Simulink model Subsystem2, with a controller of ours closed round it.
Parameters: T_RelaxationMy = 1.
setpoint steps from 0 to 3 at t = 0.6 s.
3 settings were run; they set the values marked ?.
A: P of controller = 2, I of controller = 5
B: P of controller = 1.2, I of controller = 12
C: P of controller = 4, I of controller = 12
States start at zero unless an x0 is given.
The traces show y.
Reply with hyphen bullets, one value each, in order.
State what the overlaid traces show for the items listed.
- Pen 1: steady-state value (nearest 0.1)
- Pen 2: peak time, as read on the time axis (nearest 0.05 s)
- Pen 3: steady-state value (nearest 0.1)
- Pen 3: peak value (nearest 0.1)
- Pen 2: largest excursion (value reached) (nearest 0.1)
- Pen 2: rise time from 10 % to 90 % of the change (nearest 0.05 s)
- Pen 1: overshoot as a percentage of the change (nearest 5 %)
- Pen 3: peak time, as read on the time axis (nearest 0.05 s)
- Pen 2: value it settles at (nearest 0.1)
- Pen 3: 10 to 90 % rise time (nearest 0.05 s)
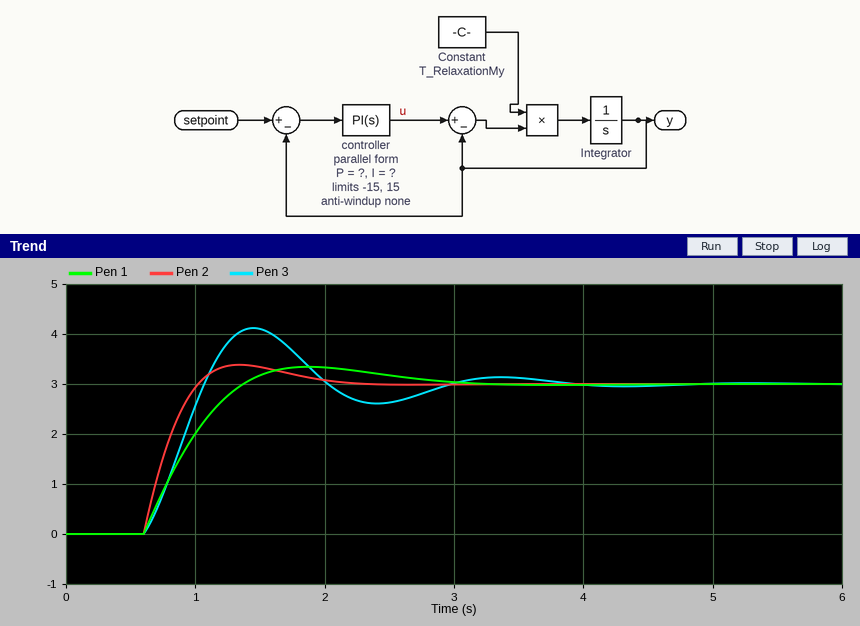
- 3.0
- 1.35 s
- 3.0
- 4.1
- 3.4
- 0.30 s
- 10 %
- 1.45 s
- 3.0
- 0.35 s
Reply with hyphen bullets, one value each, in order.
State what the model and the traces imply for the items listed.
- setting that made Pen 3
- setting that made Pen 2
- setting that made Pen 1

- B
- C
- A
